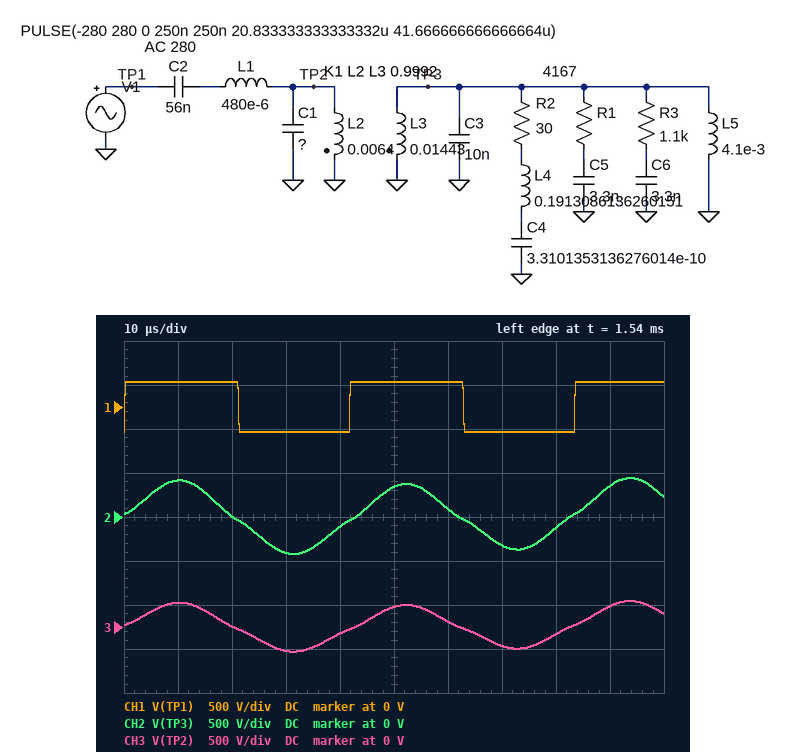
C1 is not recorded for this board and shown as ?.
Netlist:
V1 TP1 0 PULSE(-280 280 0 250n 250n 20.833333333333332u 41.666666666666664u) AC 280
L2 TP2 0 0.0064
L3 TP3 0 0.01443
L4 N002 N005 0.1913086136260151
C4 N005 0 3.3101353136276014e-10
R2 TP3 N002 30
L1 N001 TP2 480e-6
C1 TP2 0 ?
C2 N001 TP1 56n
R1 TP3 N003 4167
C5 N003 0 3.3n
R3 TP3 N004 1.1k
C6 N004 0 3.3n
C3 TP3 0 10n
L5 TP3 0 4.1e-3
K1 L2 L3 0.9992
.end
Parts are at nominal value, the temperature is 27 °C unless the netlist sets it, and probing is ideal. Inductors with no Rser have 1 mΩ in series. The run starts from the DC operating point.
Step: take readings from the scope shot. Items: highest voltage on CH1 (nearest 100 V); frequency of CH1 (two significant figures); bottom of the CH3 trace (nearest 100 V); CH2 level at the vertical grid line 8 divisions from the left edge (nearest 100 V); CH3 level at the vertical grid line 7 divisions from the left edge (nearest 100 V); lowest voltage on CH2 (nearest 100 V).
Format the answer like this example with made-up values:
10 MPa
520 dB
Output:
300 V
24 kHz
-300 V
-100 V
-200 V
-400 V
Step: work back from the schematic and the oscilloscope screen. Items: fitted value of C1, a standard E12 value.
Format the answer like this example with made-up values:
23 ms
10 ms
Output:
68 nF
